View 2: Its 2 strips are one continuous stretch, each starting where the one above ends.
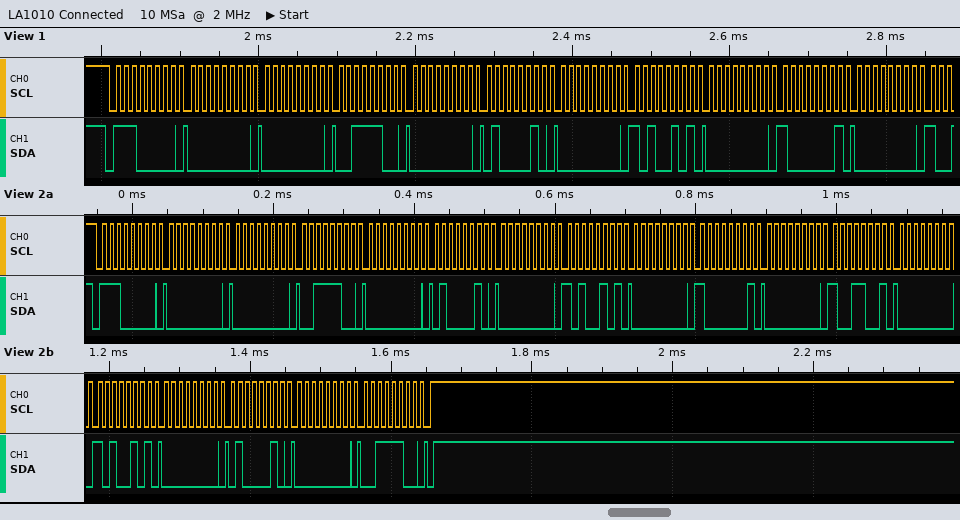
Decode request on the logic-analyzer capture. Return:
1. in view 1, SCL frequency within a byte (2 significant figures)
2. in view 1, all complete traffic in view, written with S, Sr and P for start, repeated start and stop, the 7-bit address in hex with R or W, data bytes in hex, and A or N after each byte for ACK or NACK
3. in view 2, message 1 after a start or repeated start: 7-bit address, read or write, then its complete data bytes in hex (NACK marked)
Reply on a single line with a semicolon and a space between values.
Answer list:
100 kHz; S 70W A 00 A 00 A 3C A 00 A 42 A 00 A A5 A 00 A 81 A 00 A; 0x70 write: 00 00 3C 00 42 00 A5 00 81 00 99 00 A5 00 42 00 3C
